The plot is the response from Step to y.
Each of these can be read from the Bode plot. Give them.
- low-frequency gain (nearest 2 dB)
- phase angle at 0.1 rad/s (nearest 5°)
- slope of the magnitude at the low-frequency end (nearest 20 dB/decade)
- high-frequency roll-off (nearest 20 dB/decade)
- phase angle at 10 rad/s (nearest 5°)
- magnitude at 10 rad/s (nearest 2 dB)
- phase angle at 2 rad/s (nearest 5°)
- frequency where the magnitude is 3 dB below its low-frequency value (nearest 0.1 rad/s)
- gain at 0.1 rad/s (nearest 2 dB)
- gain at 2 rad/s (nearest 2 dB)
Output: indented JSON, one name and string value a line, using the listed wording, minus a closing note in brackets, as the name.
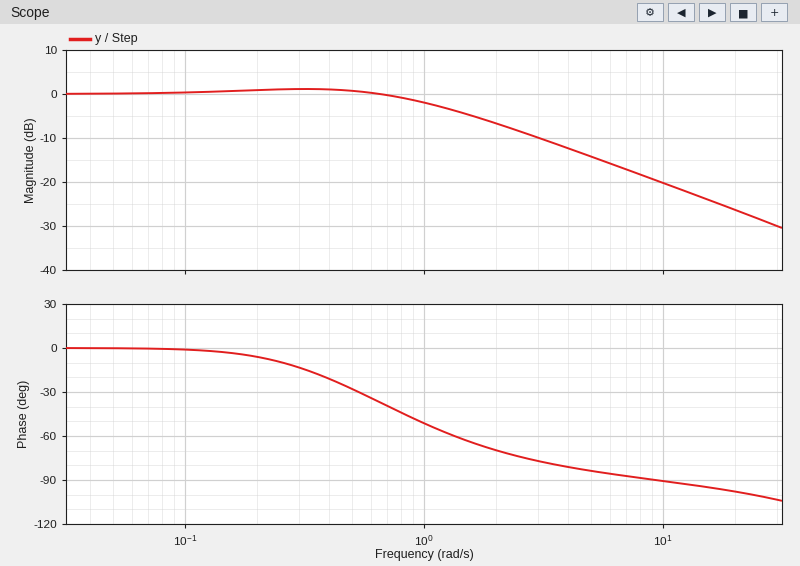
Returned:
{
  "low-frequency gain": "0 dB",
  "phase angle at 0.1 rad/s": "0°",
  "slope of the magnitude at the low-frequency end": "0 dB/decade",
  "high-frequency roll-off": "-20 dB/decade",
  "phase angle at 10 rad/s": "-90°",
  "magnitude at 10 rad/s": "-20 dB",
  "phase angle at 2 rad/s": "-70°",
  "frequency where the magnitude is 3 dB below its low-frequency value": "1.2 rad/s",
  "gain at 0.1 rad/s": "0 dB",
  "gain at 2 rad/s": "-6 dB"
}
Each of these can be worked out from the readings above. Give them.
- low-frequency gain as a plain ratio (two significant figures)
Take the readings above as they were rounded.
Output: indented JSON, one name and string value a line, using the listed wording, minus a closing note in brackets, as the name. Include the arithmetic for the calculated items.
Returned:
{
  "low-frequency gain as a plain ratio": "10^(0 / 20) = 1.0"
}
